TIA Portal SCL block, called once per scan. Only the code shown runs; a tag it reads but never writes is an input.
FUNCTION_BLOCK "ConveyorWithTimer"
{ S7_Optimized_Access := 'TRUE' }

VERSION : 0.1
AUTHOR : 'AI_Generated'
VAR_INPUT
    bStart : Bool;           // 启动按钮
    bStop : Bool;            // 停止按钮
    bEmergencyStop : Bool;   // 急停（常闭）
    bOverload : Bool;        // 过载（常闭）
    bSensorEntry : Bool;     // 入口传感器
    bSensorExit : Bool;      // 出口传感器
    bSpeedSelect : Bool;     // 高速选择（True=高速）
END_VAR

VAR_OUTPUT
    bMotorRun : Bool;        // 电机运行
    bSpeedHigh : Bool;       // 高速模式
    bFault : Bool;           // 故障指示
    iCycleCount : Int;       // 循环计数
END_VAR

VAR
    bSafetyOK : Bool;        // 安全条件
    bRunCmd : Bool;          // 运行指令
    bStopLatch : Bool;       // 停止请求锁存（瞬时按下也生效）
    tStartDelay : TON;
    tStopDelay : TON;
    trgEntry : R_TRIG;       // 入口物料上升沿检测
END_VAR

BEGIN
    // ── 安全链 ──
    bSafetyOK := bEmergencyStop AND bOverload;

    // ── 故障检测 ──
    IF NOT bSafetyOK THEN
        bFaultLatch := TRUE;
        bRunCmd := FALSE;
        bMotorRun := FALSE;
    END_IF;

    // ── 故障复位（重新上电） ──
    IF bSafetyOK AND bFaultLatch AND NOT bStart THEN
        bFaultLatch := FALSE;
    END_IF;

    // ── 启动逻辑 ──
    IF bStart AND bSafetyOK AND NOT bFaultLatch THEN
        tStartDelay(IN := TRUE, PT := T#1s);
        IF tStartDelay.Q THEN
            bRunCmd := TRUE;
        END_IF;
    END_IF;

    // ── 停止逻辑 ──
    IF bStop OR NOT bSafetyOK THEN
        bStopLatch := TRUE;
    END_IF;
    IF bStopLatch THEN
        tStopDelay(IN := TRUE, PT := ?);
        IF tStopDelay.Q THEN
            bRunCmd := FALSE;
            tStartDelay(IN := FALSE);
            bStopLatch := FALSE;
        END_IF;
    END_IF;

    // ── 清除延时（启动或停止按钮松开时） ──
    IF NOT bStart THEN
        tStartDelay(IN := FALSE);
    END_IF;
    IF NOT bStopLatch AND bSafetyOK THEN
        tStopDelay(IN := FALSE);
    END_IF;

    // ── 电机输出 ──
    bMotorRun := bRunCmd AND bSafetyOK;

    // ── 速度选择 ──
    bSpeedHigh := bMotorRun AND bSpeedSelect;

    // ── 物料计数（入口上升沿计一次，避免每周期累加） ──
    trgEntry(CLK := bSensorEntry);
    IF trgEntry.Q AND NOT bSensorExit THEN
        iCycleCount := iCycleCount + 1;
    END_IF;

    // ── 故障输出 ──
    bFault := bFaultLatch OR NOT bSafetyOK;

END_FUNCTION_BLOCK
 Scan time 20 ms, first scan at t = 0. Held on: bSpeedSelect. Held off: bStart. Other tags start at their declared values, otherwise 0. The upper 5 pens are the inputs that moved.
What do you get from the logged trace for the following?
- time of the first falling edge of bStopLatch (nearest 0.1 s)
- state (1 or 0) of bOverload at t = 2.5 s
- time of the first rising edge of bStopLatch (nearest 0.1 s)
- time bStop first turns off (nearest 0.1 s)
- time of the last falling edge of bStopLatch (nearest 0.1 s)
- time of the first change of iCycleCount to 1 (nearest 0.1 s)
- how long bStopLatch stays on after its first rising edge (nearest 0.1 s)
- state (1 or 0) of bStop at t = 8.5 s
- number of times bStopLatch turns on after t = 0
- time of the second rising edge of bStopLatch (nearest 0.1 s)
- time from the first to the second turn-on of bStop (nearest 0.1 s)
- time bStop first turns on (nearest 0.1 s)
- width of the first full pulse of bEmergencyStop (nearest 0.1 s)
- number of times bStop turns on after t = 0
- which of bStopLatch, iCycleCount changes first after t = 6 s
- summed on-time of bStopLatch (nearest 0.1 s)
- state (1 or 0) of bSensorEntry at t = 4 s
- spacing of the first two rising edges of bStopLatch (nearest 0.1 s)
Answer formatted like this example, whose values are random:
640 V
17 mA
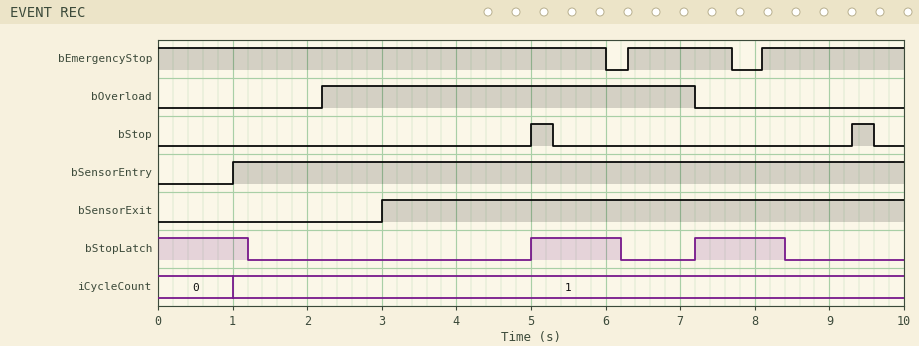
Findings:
1.2 s
1
5.0 s
5.3 s
8.4 s
1.0 s
1.2 s
0
2
7.2 s
4.3 s
5.0 s
1.4 s
2
bStopLatch
3.6 s
1
2.2 s
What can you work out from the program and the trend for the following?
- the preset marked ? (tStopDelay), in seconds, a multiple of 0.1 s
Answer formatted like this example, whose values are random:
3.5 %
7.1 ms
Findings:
1.2 s
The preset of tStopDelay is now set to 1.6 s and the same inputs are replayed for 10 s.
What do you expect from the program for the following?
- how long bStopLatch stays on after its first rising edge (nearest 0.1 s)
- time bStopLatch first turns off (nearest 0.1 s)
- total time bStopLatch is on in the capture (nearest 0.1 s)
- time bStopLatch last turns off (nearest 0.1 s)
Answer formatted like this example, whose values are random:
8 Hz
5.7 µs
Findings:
1.6 s
1.6 s
4.8 s
8.8 s
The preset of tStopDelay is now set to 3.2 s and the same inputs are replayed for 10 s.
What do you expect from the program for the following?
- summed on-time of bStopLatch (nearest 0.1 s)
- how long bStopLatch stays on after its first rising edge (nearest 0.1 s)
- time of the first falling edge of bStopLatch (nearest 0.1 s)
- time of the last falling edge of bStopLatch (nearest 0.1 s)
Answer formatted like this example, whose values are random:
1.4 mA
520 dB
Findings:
6.4 s
3.2 s
3.2 s
8.2 s
